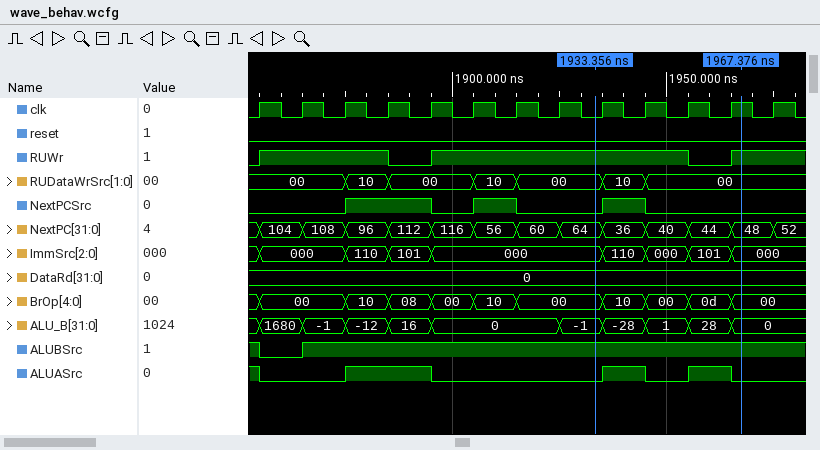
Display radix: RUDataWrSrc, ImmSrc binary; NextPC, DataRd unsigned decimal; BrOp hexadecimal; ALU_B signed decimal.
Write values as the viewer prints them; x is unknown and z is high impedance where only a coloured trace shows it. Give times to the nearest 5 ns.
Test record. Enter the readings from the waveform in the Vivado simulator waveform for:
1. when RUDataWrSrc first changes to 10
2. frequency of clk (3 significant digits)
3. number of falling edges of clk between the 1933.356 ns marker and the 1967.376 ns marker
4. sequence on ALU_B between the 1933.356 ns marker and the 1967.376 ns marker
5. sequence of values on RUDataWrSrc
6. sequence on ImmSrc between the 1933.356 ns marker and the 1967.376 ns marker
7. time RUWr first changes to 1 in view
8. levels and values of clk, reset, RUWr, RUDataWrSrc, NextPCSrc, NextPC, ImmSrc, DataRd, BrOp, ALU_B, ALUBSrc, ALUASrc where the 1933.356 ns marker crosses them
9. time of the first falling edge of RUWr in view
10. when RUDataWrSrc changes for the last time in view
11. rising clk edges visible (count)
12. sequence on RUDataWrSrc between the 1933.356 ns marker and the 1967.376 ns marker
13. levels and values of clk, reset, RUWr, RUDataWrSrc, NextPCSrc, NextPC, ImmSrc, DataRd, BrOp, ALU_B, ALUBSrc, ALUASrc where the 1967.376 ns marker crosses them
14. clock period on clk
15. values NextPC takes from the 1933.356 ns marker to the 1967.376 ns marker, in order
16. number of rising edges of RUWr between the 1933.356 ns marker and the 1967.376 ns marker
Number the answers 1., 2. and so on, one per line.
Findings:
1. 1875 ns
2. 100 MHz
3. 3
4. -1, -28, 1, 28, 0
5. 00, 10, 00, 10, 00, 10, 00
6. 000, 110, 000, 101, 000
7. 1855 ns
8. clk=0, reset=0, RUWr=1, RUDataWrSrc=00, NextPCSrc=0, NextPC=64, ImmSrc=000, DataRd=0, BrOp=00, ALU_B=-1, ALUBSrc=1, ALUASrc=0
9. 1885 ns
10. 1945 ns
11. 13
12. 00, 10, 00
13. clk=1, reset=0, RUWr=1, RUDataWrSrc=00, NextPCSrc=0, NextPC=48, ImmSrc=000, DataRd=0, BrOp=00, ALU_B=0, ALUBSrc=1, ALUASrc=0
14. 10 ns
15. 64, 36, 40, 44, 48
16. 1
